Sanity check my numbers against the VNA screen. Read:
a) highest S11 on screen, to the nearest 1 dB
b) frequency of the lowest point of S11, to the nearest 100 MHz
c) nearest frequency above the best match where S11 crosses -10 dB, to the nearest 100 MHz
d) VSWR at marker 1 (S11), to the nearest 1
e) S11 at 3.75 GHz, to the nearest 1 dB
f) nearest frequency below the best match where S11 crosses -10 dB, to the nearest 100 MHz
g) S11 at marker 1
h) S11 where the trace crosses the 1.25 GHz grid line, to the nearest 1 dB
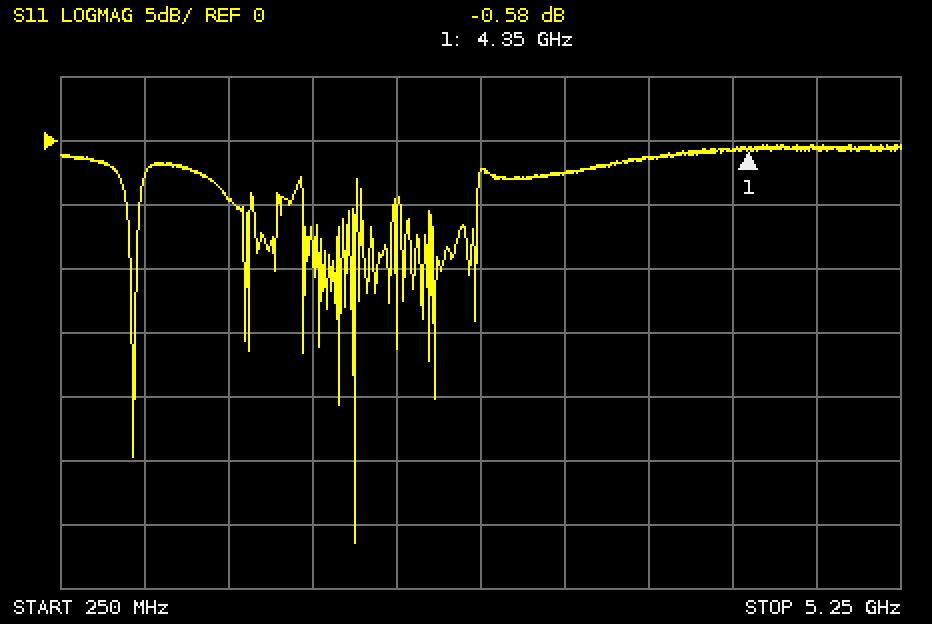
0 dB
2.0 GHz
2.0 GHz
30
-1 dB
2.0 GHz
-0.58 dB
-5 dB
